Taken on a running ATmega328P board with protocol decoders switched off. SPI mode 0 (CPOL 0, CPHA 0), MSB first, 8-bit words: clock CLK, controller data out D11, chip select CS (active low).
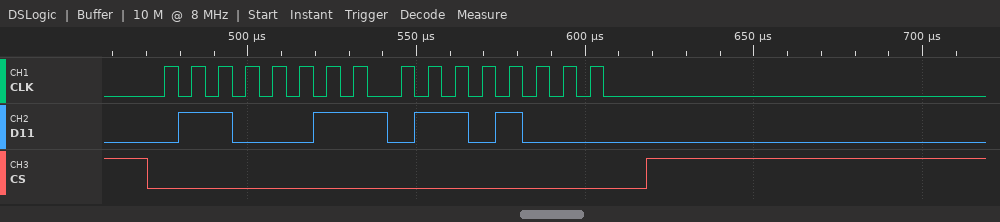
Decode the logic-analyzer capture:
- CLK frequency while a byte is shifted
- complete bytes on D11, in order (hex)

125 kHz
63 68
